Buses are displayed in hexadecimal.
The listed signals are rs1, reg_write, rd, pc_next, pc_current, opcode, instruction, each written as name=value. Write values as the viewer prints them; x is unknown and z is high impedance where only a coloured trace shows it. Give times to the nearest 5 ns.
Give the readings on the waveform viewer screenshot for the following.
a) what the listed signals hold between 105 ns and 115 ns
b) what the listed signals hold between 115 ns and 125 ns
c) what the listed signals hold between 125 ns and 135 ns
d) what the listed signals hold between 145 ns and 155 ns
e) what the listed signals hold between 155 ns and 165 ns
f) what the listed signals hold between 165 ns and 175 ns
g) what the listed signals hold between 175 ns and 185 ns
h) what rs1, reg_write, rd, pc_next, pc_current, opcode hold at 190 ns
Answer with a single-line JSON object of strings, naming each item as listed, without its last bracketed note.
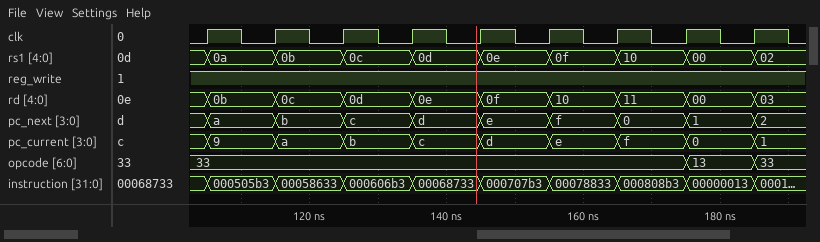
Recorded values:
{"what the listed signals hold between 105 ns and 115 ns": "rs1=0a, reg_write=1, rd=0b, pc_next=a, pc_current=9, opcode=33, instruction=000505b3", "what the listed signals hold between 115 ns and 125 ns": "rs1=0b, reg_write=1, rd=0c, pc_next=b, pc_current=a, opcode=33, instruction=00058633", "what the listed signals hold between 125 ns and 135 ns": "rs1=0c, reg_write=1, rd=0d, pc_next=c, pc_current=b, opcode=33, instruction=000606b3", "what the listed signals hold between 145 ns and 155 ns": "rs1=0e, reg_write=1, rd=0f, pc_next=e, pc_current=d, opcode=33, instruction=000707b3", "what the listed signals hold between 155 ns and 165 ns": "rs1=0f, reg_write=1, rd=10, pc_next=f, pc_current=e, opcode=33, instruction=00078833", "what the listed signals hold between 165 ns and 175 ns": "rs1=10, reg_write=1, rd=11, pc_next=0, pc_current=f, opcode=33, instruction=000808b3", "what the listed signals hold between 175 ns and 185 ns": "rs1=00, reg_write=1, rd=00, pc_next=1, pc_current=0, opcode=13, instruction=00000013", "what rs1, reg_write, rd, pc_next, pc_current, opcode hold at 190 ns": "rs1=02, reg_write=1, rd=03, pc_next=2, pc_current=1, opcode=33"}
